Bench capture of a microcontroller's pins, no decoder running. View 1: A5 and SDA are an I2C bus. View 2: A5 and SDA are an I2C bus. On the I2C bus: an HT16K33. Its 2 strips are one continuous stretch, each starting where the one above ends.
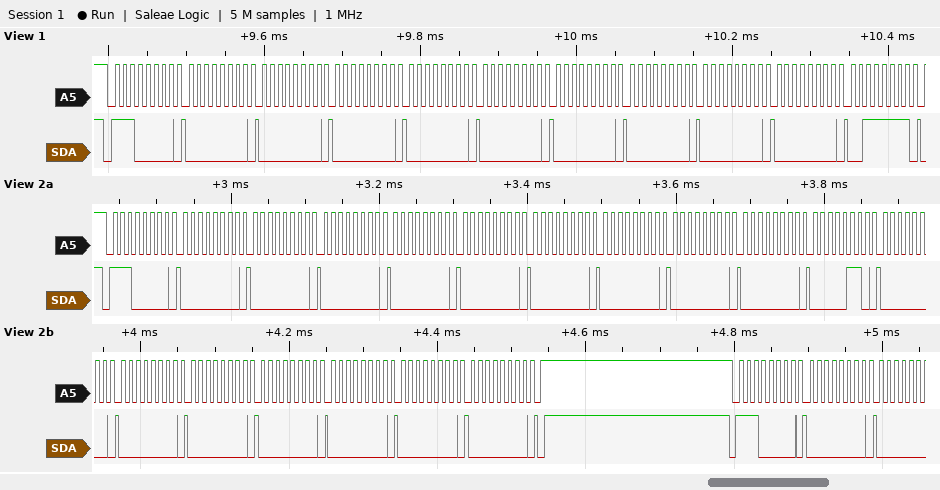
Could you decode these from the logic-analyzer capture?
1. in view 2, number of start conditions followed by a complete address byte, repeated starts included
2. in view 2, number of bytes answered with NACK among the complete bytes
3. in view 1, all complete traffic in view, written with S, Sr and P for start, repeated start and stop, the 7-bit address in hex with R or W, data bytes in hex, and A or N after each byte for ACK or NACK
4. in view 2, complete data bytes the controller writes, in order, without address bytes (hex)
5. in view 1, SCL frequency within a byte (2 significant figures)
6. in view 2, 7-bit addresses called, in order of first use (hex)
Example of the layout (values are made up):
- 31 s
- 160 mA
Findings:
- 2
- 0
- S 70W A 00 A 00 A 00 A 00 A 00 A 00 A 00 A 00 A 00 A 3F A
- 00 00 00 00 00 00 00 00 00 06 00 00 00 00 00 00 00 00
- 100 kHz
- 0x70
